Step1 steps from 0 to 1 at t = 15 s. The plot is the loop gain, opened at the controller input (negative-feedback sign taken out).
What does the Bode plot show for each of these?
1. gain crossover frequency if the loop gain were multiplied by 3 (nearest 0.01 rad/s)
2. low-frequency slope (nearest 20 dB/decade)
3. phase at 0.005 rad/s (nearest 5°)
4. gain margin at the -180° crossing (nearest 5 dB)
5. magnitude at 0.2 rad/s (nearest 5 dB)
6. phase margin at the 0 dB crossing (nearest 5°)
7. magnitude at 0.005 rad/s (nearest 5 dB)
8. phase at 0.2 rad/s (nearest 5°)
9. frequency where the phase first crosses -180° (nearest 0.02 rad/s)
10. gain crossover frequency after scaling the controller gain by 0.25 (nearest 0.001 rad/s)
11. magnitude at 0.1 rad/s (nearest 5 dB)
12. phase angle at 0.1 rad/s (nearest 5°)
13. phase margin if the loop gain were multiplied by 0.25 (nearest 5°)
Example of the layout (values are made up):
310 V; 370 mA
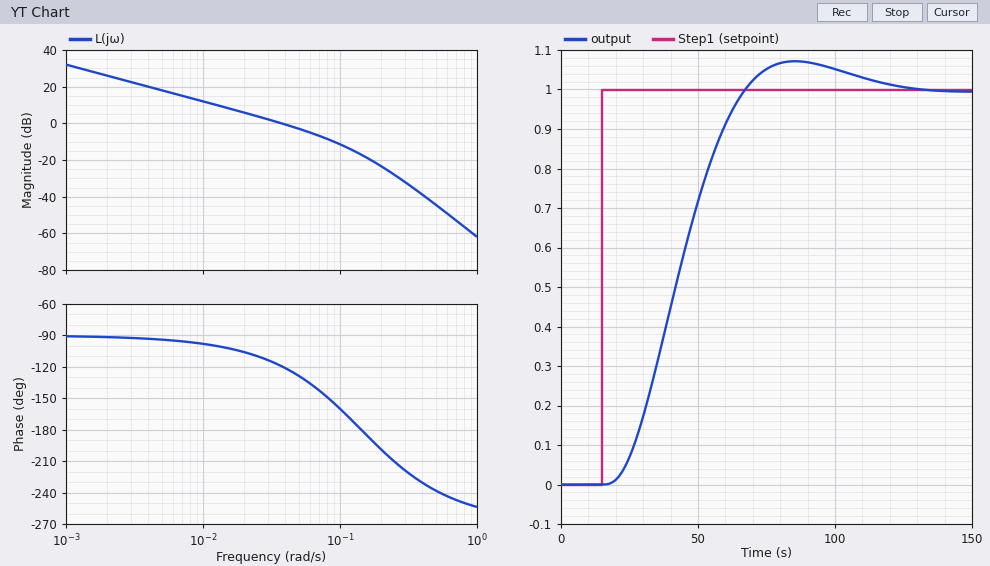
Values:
0.09 rad/s; -20 dB/decade; -95°; 15 dB; -25 dB; 60°; 20 dB; -200°; 0.14 rad/s; 0.010 rad/s; -10 dB; -160°; 80°
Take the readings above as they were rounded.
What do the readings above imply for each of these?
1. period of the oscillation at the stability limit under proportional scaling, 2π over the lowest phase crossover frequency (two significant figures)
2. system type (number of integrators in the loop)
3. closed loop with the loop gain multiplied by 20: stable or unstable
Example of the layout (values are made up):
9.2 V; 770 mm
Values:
45 s; 1; unstable
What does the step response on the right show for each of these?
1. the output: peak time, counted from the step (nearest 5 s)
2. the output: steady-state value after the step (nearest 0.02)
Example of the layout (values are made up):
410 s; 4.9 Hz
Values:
70 s; 1.00
